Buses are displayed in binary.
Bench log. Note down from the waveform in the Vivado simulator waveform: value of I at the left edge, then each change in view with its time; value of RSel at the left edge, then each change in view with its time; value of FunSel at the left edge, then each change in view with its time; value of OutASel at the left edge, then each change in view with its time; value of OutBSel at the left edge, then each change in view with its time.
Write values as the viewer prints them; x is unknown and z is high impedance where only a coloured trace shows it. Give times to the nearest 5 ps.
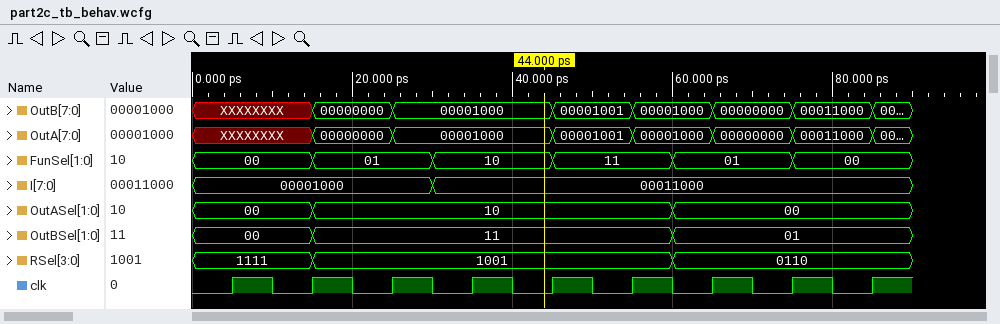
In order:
00001000, 00011000 at 30 ps
1111, 1001 at 15 ps, 0110 at 60 ps
00, 01 at 15 ps, 10 at 30 ps, 11 at 45 ps, 01 at 60 ps, 00 at 75 ps
00, 10 at 15 ps, 00 at 60 ps
00, 11 at 15 ps, 01 at 60 ps
